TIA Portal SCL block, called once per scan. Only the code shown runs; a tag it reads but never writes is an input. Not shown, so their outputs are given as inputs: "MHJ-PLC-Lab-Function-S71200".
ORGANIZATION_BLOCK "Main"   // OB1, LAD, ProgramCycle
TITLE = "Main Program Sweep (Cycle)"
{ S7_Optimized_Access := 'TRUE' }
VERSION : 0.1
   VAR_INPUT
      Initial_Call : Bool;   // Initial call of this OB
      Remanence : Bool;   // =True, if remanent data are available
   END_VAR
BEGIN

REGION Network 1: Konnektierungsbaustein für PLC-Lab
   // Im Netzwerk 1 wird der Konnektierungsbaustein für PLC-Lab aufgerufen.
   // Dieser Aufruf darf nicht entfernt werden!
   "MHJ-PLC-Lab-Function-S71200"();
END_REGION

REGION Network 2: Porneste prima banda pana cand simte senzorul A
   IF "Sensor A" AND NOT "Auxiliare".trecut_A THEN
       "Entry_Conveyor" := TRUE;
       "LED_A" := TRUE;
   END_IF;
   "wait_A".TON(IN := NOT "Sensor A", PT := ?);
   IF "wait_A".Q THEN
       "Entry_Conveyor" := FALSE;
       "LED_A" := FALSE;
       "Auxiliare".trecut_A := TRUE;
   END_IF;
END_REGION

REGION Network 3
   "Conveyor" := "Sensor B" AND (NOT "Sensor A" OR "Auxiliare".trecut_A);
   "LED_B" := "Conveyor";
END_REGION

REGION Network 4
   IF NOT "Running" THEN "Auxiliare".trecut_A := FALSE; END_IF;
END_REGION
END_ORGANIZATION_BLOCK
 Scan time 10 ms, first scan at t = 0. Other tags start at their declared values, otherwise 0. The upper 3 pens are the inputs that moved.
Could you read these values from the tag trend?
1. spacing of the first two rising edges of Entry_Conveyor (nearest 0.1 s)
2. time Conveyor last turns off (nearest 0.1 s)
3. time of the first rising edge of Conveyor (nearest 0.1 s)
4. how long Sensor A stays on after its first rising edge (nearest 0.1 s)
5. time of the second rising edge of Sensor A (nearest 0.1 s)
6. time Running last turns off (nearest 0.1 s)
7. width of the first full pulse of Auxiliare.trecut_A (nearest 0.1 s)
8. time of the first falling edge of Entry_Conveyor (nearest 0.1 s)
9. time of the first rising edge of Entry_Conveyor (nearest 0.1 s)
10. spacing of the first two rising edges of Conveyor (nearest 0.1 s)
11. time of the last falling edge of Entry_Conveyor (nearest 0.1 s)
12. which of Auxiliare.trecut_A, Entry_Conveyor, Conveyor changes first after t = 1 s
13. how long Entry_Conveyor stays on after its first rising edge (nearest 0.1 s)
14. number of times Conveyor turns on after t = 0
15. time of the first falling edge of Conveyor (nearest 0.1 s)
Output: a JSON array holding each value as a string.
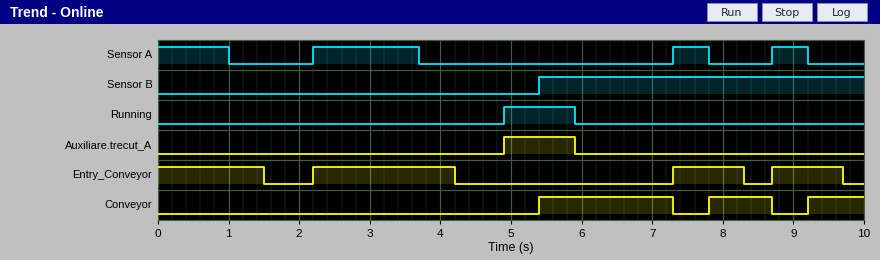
["5.1 s", "8.7 s", "5.4 s", "1.5 s", "7.3 s", "5.9 s", "1.0 s", "1.5 s", "2.2 s", "2.4 s", "9.7 s", "Entry_Conveyor", "2.0 s", "3", "7.3 s"]
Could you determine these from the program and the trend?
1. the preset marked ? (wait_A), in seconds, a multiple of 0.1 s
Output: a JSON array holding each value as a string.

["0.5 s"]
